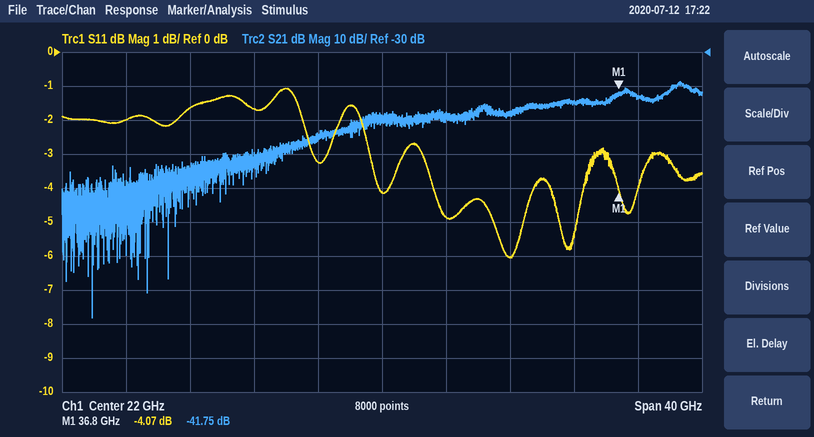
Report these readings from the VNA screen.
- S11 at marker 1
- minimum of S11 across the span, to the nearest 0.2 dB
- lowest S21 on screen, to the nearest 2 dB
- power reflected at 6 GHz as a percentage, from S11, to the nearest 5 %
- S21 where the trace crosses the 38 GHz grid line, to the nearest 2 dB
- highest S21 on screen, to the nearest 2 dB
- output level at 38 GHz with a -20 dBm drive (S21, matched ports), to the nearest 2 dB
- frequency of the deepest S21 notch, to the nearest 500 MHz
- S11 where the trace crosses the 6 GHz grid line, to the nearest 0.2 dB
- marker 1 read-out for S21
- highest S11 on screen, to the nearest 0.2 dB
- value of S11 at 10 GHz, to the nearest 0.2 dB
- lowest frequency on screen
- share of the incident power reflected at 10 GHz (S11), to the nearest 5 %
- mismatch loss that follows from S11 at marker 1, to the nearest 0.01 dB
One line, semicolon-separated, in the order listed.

-4.07 dB; -6.0 dB; -108 dB; 65 %; -44 dB; -38 dB; -64 dBm; 4.0 GHz; -2.0 dB; -41.75 dB; -1.0 dB; -1.6 dB; 2 GHz; 70 %; 2.16 dB
